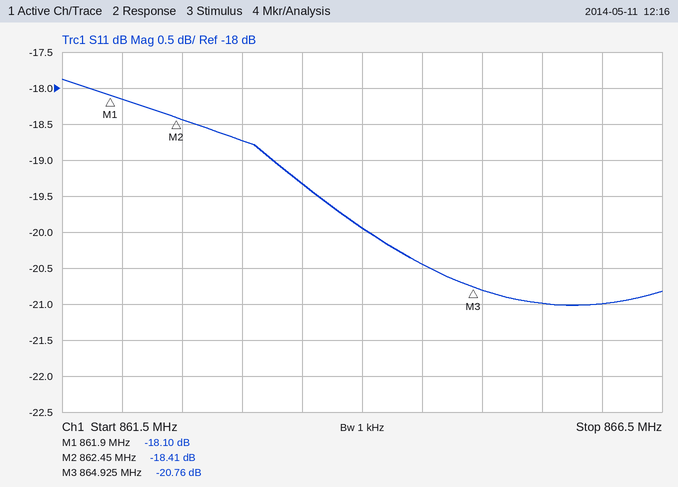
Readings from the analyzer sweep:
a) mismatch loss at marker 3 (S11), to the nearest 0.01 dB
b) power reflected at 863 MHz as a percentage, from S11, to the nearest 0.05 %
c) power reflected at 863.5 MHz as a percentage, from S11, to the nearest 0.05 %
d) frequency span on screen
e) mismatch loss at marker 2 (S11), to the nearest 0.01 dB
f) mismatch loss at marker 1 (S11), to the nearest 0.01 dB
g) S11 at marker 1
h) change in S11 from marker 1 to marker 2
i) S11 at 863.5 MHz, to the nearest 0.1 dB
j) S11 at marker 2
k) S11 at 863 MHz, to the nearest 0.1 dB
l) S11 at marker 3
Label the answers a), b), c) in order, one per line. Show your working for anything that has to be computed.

a) −10 log10(1 − 10^(-20.76/10)) ≈ 0.04 dB
b) 10^(-18.7/10) ≈ 1.35 %
c) 10^(-19.3/10) ≈ 1.17 %, so 1.15 % to the nearest 0.05 %
d) 5 MHz
e) −10 log10(1 − 10^(-18.41/10)) ≈ 0.06 dB
f) −10 log10(1 − 10^(-18.1/10)) ≈ 0.07 dB
g) -18.10 dB
h) -18.41 − (-18.1) = -0.31 dB
i) -19.3 dB
j) -18.41 dB
k) -18.7 dB
l) -20.76 dB
